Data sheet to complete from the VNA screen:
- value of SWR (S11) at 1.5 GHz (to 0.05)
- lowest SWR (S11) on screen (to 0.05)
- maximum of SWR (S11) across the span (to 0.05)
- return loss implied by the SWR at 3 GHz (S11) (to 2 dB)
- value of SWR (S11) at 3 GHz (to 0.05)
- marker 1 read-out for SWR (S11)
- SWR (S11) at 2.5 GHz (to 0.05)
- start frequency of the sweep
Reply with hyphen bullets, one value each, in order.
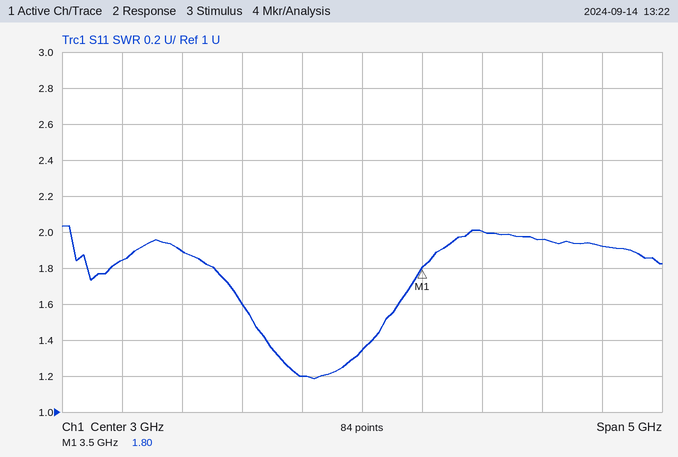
- 1.90
- 1.20
- 2.05
- 16 dB
- 1.35
- 1.80
- 1.20
- 500 MHz
